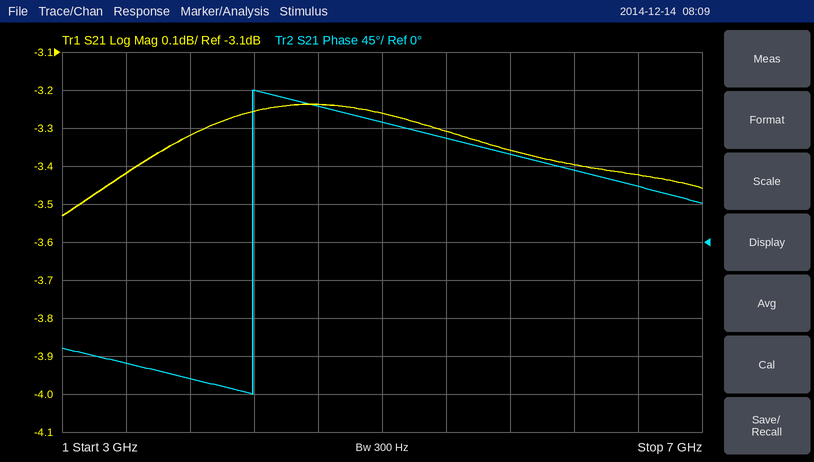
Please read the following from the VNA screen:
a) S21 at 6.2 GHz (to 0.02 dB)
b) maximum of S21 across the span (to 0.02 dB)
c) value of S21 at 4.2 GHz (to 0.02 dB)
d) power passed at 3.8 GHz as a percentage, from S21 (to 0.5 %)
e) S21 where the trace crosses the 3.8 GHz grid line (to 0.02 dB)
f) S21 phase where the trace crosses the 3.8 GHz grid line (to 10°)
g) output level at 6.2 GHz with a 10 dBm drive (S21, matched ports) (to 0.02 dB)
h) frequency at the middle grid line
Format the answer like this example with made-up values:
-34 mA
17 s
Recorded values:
-3.40 dB
-3.24 dB
-3.26 dB
46.5 %
-3.32 dB
-160°
6.60 dBm
5 GHz
